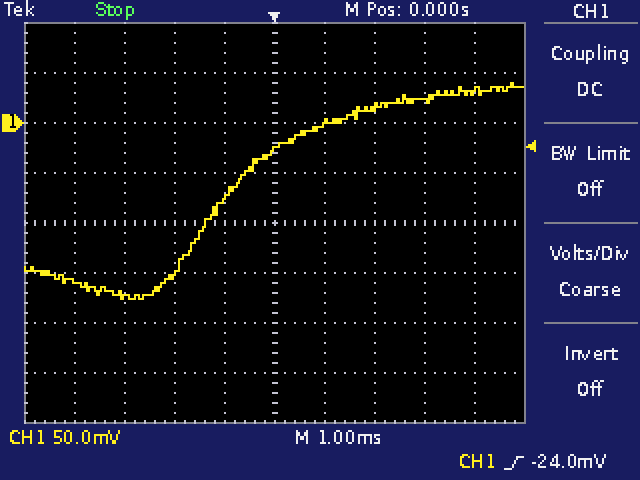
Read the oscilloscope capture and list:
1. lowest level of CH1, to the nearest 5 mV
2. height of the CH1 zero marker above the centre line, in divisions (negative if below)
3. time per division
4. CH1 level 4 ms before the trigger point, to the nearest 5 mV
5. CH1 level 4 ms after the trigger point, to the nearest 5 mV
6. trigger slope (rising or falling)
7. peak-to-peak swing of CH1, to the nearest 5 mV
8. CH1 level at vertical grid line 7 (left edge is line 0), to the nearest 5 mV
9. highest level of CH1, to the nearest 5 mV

-175 mV
+2.0 div
1 ms
-160 mV
30 mV
rising
215 mV
15 mV
40 mV
